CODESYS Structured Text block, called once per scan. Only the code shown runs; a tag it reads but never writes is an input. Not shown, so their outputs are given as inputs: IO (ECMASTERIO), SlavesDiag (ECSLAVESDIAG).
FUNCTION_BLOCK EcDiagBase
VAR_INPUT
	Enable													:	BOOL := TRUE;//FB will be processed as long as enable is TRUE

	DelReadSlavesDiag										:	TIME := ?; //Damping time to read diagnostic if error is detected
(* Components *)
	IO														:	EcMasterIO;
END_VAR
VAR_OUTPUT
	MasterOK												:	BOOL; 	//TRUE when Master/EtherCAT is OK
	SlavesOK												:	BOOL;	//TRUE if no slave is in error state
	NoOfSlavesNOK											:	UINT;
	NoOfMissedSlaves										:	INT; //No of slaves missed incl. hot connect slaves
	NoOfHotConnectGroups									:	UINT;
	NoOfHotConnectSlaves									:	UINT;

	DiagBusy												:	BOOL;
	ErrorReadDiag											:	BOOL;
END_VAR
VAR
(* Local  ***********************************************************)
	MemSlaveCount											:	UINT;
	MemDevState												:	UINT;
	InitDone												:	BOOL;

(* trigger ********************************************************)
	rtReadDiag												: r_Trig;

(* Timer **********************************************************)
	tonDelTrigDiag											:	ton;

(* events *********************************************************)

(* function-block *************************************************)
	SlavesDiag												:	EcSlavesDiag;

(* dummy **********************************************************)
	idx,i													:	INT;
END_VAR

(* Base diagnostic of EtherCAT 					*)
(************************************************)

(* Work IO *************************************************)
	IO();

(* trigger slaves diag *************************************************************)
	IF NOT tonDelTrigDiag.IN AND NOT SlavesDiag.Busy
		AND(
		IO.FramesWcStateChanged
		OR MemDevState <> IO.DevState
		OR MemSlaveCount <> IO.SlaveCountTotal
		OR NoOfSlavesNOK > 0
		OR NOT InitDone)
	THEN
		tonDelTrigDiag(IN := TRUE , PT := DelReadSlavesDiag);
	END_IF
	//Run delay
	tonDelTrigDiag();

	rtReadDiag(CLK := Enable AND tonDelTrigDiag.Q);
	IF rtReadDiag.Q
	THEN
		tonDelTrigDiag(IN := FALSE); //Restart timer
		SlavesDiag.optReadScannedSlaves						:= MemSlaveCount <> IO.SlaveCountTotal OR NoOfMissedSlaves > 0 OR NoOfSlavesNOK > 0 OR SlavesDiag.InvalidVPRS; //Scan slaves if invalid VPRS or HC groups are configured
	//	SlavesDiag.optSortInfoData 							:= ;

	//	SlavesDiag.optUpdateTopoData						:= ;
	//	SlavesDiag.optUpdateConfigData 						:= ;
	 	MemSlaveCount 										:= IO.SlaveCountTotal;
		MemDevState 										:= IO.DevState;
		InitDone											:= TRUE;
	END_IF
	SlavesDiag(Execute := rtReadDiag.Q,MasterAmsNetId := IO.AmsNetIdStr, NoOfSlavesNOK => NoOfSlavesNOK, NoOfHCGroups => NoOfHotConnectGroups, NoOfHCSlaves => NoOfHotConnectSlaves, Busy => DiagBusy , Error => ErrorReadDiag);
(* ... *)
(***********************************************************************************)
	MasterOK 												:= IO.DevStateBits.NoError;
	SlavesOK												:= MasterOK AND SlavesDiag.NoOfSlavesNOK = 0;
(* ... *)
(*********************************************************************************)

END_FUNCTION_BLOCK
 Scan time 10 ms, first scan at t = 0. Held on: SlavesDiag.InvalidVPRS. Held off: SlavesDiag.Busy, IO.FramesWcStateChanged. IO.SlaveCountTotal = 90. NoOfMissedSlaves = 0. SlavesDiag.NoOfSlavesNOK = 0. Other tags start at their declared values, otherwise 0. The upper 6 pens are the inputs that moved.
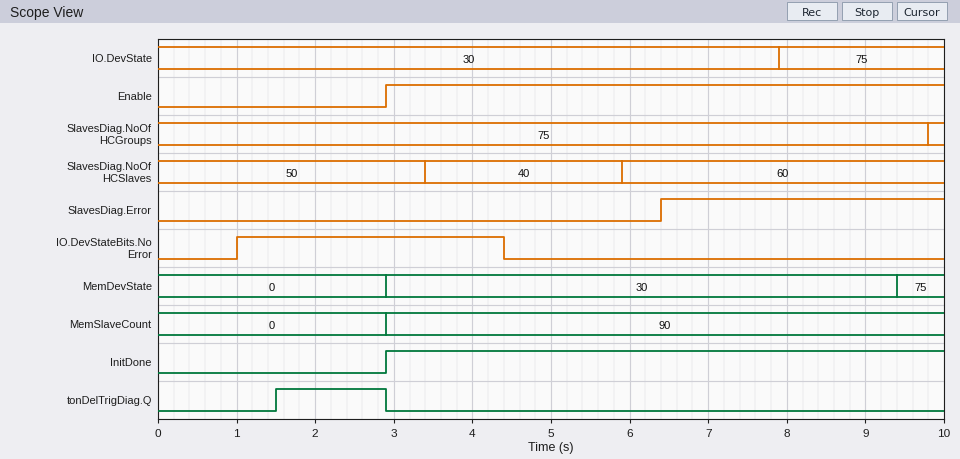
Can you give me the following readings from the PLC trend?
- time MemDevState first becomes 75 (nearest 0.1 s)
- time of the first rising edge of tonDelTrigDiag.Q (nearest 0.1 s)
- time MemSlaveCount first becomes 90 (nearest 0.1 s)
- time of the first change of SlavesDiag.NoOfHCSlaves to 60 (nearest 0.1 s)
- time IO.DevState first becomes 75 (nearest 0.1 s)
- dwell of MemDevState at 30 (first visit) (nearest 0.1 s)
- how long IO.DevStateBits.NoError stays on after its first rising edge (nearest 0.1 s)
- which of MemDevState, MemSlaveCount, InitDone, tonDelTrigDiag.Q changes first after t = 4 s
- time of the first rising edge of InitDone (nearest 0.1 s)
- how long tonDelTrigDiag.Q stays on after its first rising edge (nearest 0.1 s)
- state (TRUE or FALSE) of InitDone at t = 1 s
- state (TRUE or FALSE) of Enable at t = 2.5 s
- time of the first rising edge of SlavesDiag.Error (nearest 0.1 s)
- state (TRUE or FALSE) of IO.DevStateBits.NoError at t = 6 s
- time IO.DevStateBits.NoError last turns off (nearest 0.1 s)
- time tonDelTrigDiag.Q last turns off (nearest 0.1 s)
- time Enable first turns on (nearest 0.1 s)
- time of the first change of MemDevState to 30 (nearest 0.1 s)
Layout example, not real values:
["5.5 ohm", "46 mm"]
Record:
["9.4 s", "1.5 s", "2.9 s", "5.9 s", "7.9 s", "6.5 s", "3.4 s", "MemDevState", "2.9 s", "1.4 s", "FALSE", "FALSE", "6.4 s", "FALSE", "4.4 s", "2.9 s", "2.9 s", "2.9 s"]
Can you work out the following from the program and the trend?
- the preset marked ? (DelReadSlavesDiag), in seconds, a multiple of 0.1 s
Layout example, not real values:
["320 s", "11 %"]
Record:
["1.5 s"]
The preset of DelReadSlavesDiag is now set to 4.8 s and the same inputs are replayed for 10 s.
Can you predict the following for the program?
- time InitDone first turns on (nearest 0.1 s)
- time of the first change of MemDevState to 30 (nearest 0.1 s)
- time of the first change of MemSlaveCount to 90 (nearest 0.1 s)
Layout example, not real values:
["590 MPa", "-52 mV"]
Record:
["4.8 s", "4.8 s", "4.8 s"]
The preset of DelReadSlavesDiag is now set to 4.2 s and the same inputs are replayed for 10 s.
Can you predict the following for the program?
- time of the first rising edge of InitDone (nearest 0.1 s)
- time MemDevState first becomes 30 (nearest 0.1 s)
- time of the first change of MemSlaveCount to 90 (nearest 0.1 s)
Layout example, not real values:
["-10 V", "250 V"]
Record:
["4.2 s", "4.2 s", "4.2 s"]
